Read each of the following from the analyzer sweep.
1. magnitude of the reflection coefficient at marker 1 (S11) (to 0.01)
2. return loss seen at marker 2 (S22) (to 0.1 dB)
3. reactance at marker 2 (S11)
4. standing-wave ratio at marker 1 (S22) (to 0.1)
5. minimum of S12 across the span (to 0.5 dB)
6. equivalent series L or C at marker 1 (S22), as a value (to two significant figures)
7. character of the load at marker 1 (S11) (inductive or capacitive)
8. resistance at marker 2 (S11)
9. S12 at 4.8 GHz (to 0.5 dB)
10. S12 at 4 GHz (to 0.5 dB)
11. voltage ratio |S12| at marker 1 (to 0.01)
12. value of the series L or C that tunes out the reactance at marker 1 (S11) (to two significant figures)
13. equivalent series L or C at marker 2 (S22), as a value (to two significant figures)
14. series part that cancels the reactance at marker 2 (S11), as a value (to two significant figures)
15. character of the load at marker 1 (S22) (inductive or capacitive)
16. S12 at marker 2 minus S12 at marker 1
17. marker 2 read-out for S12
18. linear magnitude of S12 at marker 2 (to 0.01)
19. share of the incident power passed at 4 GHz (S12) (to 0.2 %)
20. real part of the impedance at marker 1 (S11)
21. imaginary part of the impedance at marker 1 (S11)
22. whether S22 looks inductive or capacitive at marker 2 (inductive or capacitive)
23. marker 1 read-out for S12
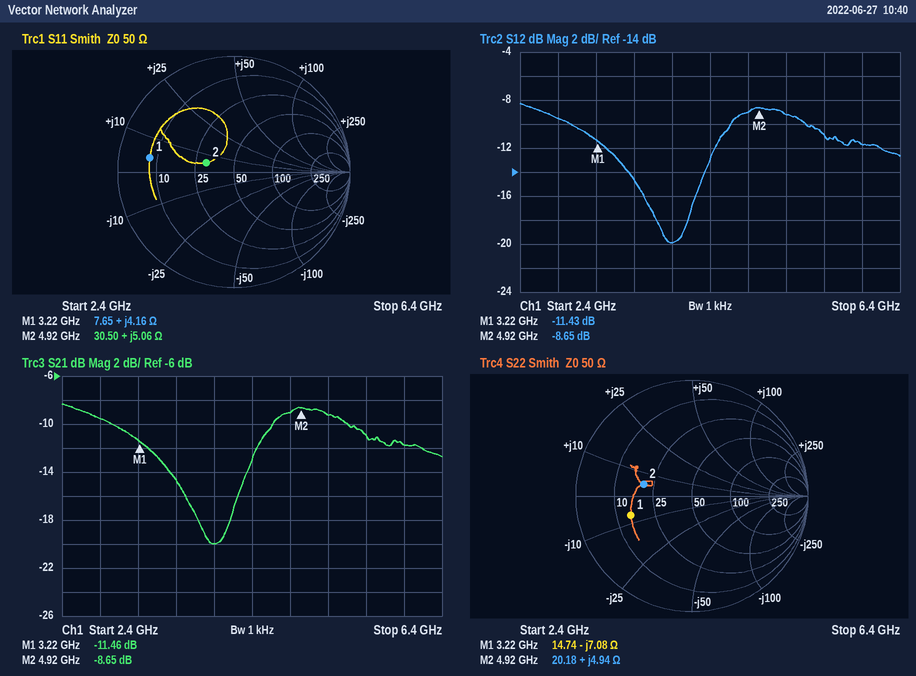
0.74
7.3 dB
+5.06 Ω
3.5
-20.0 dB
7.0 pF
inductive
30.50 Ω
-9.0 dB
-20.0 dB
0.27
12 pF
160 pH
6.4 pF
capacitive
2.78 dB
-8.65 dB
0.37
1.0 %
7.65 Ω
+4.16 Ω
inductive
-11.43 dB
